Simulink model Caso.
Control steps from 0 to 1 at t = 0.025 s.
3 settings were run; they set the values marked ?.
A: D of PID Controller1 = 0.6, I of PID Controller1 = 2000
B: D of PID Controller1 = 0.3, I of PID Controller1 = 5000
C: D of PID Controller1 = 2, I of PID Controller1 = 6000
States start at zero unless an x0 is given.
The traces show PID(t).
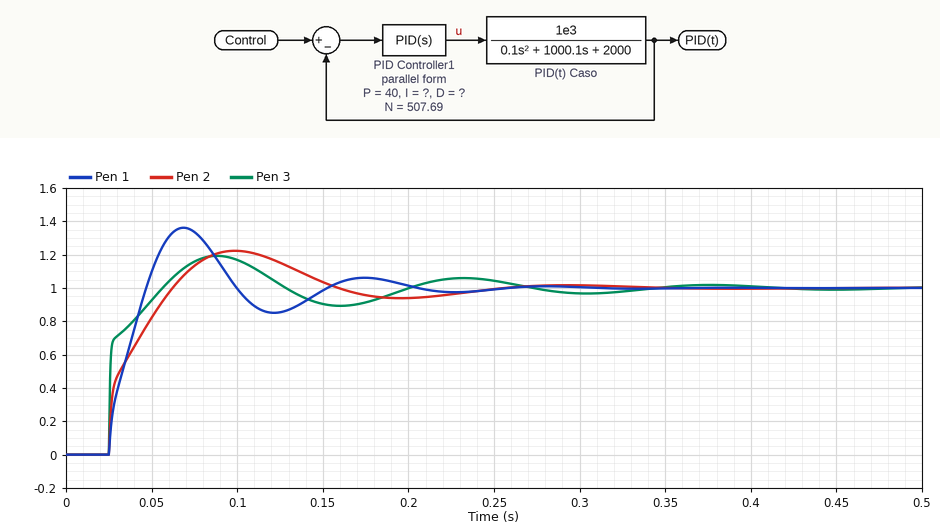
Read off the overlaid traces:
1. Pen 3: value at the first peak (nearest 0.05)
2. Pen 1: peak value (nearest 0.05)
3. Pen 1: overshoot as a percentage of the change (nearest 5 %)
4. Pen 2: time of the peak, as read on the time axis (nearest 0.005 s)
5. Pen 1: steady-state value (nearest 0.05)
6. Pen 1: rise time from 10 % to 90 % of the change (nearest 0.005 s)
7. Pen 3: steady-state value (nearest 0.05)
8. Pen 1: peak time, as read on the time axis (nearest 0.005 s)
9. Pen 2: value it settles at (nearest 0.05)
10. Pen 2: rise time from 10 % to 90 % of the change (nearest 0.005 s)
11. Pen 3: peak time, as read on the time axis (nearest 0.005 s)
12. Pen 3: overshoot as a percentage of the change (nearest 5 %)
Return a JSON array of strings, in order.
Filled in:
["1.20", "1.35", "35 %", "0.100 s", "1.00", "0.020 s", "1.00", "0.070 s", "1.00", "0.030 s", "0.090 s", "20 %"]
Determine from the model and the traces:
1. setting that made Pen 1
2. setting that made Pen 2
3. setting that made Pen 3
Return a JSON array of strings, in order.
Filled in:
["B", "A", "C"]
